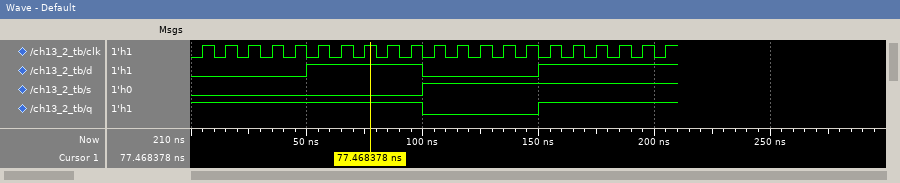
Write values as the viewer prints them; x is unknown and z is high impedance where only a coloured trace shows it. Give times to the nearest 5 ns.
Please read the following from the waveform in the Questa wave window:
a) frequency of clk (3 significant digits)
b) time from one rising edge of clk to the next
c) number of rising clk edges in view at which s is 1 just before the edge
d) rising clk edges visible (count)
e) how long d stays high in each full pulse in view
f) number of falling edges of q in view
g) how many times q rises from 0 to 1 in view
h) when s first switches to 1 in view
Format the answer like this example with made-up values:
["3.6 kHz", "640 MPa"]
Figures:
["100 MHz", "10 ns", "11", "21", "50 ns", "1", "1", "100 ns"]
